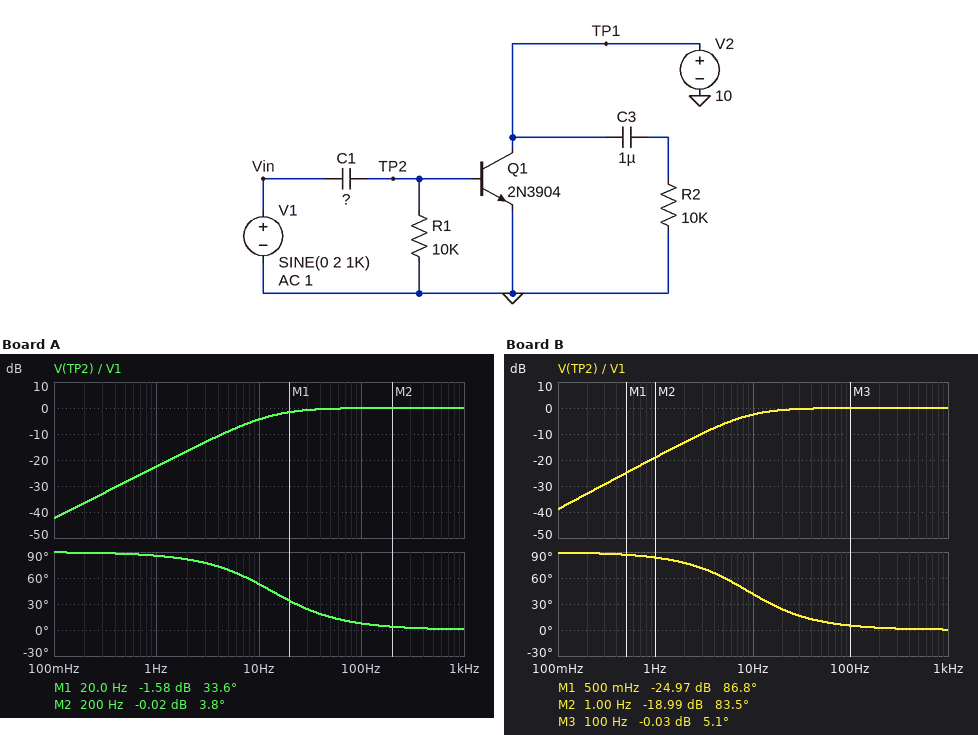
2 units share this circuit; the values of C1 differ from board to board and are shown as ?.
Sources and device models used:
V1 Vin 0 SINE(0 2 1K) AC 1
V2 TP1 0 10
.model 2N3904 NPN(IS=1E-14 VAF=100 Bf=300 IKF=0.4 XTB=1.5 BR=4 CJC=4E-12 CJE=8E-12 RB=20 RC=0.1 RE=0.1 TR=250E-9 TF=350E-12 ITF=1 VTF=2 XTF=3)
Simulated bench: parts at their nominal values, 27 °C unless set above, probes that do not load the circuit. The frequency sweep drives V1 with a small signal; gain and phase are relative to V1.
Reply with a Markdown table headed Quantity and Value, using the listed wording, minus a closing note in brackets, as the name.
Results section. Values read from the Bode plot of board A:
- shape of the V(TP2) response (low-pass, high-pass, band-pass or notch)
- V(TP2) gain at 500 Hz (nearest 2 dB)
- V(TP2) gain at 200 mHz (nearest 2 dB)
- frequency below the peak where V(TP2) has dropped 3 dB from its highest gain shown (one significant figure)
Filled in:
| Quantity | Value |
|---|---|
| shape of the V(TP2) response | high-pass |
| V(TP2) gain at 500 Hz | 0 dB |
| V(TP2) gain at 200 mHz | -36 dB |
| frequency below the peak where V(TP2) has dropped 3 dB from its highest gain shown | 10 Hz |
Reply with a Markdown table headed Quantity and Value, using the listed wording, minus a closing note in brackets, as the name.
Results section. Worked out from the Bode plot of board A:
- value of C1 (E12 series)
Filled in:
| Quantity | Value |
|---|---|
| value of C1 | 1.2 µF |
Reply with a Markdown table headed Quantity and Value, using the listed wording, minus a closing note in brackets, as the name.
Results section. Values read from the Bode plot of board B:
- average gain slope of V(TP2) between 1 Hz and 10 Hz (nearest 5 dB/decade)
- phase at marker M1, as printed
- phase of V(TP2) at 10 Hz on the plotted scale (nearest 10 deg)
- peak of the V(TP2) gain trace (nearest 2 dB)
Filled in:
| Quantity | Value |
|---|---|
| average gain slope of V(TP2) between 1 Hz and 10 Hz | 15 dB/decade |
| phase at marker M1, as printed | 86.8 deg |
| phase of V(TP2) at 10 Hz on the plotted scale | 40 deg |
| peak of the V(TP2) gain trace | 0 dB |
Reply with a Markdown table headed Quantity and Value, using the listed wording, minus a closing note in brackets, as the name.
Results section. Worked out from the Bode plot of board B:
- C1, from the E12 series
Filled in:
| Quantity | Value |
|---|---|
| C1, from the E12 series | 1.8 µF |
